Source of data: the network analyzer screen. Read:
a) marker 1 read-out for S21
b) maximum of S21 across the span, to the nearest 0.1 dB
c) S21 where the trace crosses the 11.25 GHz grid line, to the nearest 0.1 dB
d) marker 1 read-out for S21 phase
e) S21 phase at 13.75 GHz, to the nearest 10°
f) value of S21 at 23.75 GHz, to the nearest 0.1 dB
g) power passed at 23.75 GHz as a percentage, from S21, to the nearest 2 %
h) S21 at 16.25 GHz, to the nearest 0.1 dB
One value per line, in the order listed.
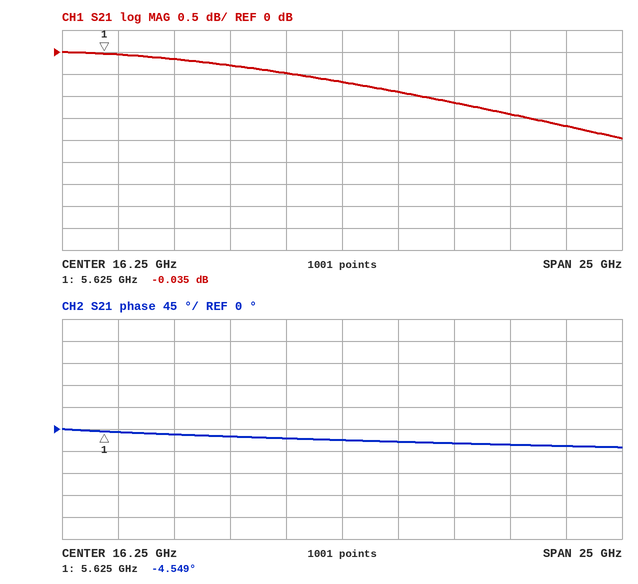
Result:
-0.035 dB
0.0 dB
-0.3 dB
-4.549°
-20°
-1.4 dB
72 %
-0.7 dB
